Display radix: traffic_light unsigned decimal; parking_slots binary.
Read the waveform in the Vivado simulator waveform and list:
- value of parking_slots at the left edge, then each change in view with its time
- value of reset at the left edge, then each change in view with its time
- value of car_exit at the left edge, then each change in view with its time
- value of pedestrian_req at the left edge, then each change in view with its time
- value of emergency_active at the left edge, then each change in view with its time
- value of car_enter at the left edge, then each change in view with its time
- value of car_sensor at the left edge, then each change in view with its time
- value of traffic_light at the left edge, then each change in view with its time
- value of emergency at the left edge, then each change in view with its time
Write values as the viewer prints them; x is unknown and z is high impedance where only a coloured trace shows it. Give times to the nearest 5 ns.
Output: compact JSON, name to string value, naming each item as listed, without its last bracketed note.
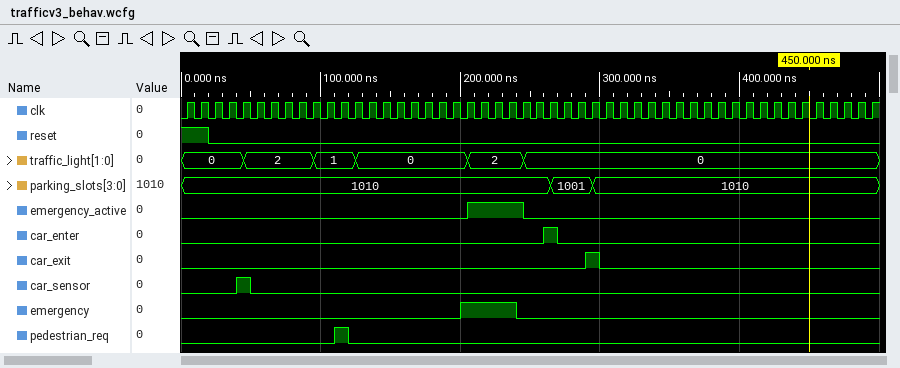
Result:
{"value of parking_slots at the left edge, then each change in view with its time": "1010, 1001 at 265 ns, 1010 at 295 ns", "value of reset at the left edge, then each change in view with its time": "1, 0 at 20 ns", "value of car_exit at the left edge, then each change in view with its time": "0, 1 at 290 ns, 0 at 300 ns", "value of pedestrian_req at the left edge, then each change in view with its time": "0, 1 at 110 ns, 0 at 120 ns", "value of emergency_active at the left edge, then each change in view with its time": "0, 1 at 205 ns, 0 at 245 ns", "value of car_enter at the left edge, then each change in view with its time": "0, 1 at 260 ns, 0 at 270 ns", "value of car_sensor at the left edge, then each change in view with its time": "0, 1 at 40 ns, 0 at 50 ns", "value of traffic_light at the left edge, then each change in view with its time": "0, 2 at 45 ns, 1 at 95 ns, 0 at 125 ns, 2 at 205 ns, 0 at 245 ns", "value of emergency at the left edge, then each change in view with its time": "0, 1 at 200 ns, 0 at 240 ns"}
